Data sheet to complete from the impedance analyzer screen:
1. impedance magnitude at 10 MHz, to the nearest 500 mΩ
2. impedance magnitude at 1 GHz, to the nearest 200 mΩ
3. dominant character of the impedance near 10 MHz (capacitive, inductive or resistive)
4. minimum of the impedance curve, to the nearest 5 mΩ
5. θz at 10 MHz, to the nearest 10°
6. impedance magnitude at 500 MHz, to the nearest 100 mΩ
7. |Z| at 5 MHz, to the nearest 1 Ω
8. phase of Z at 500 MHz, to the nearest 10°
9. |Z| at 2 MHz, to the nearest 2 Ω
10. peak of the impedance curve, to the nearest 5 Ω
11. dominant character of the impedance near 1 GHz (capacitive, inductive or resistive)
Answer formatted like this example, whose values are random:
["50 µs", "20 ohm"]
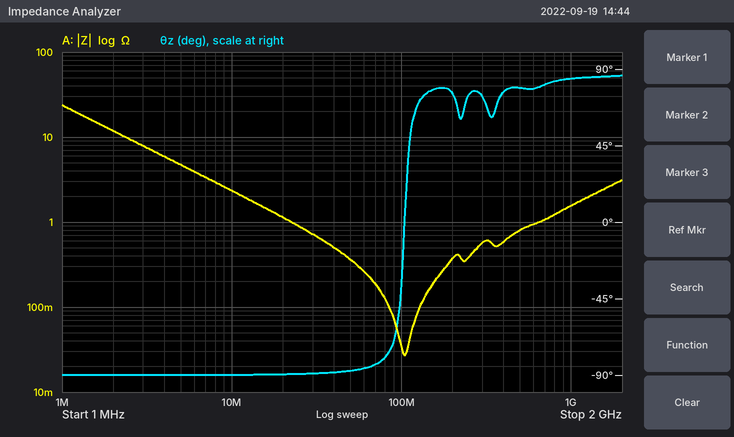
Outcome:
["2.5 Ω", "1.6 Ω", "capacitive", "25 mΩ", "-90°", "800 mΩ", "5 Ω", "80°", "12 Ω", "25 Ω", "inductive"]
